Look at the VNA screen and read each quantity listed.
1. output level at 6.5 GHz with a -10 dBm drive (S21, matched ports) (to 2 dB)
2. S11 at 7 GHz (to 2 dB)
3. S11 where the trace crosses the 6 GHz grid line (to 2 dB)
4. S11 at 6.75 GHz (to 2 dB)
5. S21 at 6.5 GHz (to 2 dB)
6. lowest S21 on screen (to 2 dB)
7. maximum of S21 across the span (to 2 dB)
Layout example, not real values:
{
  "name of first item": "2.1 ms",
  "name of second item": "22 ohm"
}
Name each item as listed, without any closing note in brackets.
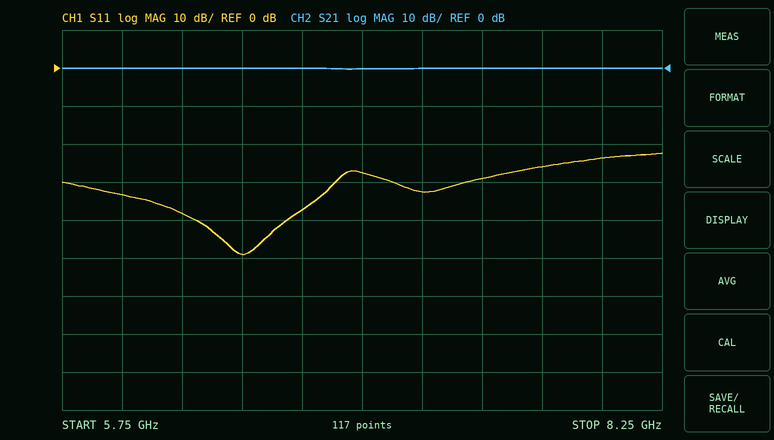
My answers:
{
  "output level at 6.5 GHz with a -10 dBm drive (S21, matched ports)": "-10 dBm",
  "S11 at 7 GHz": "-28 dB",
  "S11 where the trace crosses the 6 GHz grid line": "-34 dB",
  "S11 at 6.75 GHz": "-38 dB",
  "S21 at 6.5 GHz": "0 dB",
  "lowest S21 on screen": "0 dB",
  "maximum of S21 across the span": "0 dB"
}
